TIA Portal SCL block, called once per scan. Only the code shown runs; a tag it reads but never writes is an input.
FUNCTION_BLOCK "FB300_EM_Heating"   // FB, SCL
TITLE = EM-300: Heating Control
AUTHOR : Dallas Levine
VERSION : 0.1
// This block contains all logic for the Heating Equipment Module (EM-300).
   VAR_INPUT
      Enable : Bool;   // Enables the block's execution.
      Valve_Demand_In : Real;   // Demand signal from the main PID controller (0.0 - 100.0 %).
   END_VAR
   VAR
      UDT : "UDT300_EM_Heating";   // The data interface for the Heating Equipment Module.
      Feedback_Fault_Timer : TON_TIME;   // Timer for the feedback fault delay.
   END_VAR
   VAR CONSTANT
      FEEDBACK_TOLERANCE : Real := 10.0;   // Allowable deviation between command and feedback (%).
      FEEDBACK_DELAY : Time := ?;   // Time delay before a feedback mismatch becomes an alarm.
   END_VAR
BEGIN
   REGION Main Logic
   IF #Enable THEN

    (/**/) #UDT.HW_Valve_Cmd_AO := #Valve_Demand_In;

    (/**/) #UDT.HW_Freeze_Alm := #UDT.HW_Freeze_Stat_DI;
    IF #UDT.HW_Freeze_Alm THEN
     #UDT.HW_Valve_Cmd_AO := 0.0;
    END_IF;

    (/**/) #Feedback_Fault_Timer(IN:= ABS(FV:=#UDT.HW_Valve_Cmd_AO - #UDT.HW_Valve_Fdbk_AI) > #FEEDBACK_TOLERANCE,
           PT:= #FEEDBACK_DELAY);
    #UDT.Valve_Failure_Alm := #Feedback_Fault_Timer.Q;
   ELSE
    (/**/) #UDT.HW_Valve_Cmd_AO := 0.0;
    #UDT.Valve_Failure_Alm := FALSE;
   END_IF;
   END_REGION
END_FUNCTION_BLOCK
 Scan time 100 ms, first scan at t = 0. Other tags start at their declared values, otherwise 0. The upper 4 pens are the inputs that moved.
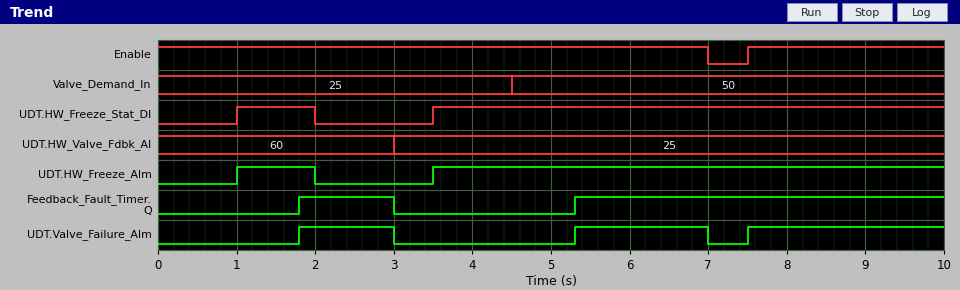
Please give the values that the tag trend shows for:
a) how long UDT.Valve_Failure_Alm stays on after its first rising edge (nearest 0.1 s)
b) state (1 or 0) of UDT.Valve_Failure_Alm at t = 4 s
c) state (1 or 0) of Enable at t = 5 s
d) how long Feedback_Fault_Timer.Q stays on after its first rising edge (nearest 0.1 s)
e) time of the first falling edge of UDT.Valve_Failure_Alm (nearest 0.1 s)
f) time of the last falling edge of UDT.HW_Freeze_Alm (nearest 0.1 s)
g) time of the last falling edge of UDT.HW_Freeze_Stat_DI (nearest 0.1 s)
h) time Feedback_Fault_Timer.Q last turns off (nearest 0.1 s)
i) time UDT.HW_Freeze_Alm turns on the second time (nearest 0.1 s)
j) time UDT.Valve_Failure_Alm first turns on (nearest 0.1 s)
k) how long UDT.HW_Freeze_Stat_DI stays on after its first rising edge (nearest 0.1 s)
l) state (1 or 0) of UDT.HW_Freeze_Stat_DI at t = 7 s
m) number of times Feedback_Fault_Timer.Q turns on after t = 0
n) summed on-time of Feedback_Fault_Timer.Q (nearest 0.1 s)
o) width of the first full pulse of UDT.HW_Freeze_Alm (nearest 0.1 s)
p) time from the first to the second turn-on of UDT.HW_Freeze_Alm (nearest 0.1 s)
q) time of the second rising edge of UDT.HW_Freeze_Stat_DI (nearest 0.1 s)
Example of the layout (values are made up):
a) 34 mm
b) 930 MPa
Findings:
a) 1.2 s
b) 0
c) 1
d) 1.2 s
e) 3.0 s
f) 2.0 s
g) 2.0 s
h) 3.0 s
i) 3.5 s
j) 1.8 s
k) 1.0 s
l) 1
m) 2
n) 5.9 s
o) 1.0 s
p) 2.5 s
q) 3.5 s
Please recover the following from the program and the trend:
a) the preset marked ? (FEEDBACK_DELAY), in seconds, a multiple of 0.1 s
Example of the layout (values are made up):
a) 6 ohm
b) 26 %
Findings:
a) 1.8 s
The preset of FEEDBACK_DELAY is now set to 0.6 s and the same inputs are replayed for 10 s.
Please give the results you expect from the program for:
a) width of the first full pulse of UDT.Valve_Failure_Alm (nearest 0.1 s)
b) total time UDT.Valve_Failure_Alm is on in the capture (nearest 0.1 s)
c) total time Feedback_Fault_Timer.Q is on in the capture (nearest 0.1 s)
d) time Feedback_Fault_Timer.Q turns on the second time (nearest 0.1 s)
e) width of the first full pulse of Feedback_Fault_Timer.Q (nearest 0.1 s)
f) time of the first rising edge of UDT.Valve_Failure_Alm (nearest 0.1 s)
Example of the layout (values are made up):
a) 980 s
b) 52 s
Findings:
a) 2.4 s
b) 7.8 s
c) 8.3 s
d) 4.1 s
e) 2.4 s
f) 0.6 s
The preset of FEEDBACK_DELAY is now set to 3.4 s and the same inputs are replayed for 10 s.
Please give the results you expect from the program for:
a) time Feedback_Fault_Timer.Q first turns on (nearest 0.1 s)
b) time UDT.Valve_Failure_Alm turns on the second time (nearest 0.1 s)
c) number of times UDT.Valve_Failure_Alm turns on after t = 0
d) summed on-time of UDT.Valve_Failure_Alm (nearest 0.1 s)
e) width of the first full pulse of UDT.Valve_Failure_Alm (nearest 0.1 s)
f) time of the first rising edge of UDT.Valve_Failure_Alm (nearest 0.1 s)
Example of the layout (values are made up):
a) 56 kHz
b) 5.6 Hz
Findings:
a) 6.9 s
b) 7.5 s
c) 2
d) 2.6 s
e) 0.1 s
f) 6.9 s
